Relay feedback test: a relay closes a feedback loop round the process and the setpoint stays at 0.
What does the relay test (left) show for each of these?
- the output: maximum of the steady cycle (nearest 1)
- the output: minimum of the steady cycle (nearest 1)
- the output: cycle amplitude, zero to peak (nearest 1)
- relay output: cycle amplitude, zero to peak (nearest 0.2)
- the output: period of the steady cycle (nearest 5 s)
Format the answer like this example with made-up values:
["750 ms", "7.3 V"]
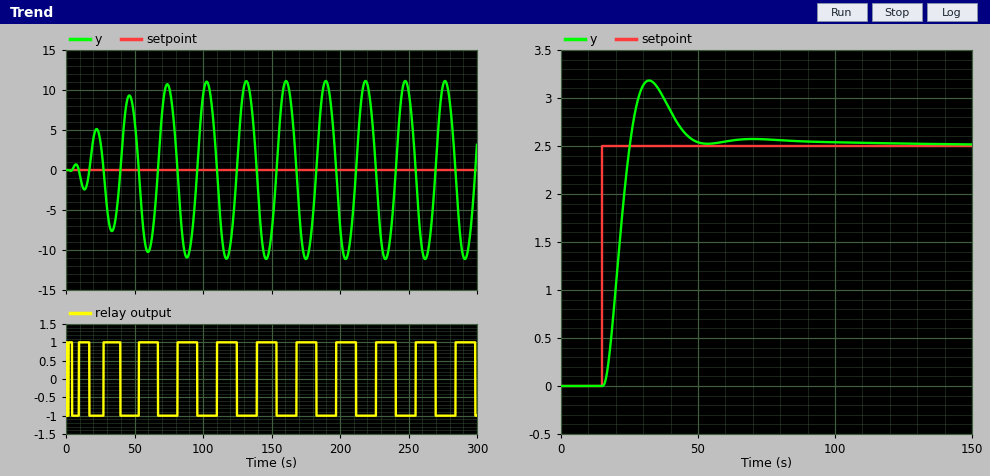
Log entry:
["11", "-11", "11", "1.0", "30 s"]
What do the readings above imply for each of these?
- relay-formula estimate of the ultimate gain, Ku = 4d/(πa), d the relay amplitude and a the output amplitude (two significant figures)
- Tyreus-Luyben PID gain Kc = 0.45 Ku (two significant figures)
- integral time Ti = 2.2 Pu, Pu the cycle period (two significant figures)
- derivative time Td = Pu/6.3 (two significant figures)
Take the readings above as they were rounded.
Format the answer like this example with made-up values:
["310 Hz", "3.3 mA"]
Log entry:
["0.12", "0.054", "66 s", "4.8 s"]
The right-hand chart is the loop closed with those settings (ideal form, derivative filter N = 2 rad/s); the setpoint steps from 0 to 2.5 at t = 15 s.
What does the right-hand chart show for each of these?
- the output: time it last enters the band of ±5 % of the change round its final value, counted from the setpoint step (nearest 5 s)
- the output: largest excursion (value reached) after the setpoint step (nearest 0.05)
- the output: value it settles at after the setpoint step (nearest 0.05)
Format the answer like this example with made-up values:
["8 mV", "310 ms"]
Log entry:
["30 s", "3.20", "2.50"]
